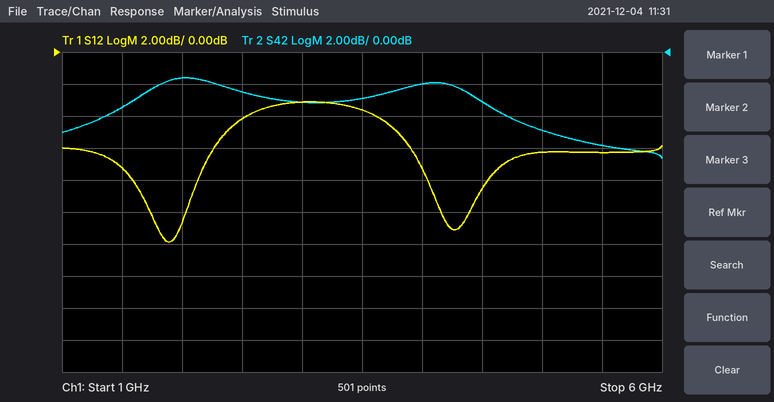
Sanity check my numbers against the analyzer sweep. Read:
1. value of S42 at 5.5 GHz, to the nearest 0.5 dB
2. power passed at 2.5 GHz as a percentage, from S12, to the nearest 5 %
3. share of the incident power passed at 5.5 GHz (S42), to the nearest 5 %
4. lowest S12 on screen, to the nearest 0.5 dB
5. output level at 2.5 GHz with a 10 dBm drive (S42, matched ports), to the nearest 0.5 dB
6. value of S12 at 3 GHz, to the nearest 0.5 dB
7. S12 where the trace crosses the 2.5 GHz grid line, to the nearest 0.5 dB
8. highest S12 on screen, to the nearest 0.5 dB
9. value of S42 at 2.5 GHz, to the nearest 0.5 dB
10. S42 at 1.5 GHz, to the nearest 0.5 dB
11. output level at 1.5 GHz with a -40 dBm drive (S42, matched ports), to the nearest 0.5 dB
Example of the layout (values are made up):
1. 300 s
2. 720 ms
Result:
1. -6.0 dB
2. 40 %
3. 25 %
4. -12.0 dB
5. 7.5 dBm
6. -3.0 dB
7. -4.0 dB
8. -3.0 dB
9. -2.5 dB
10. -3.5 dB
11. -43.5 dBm
